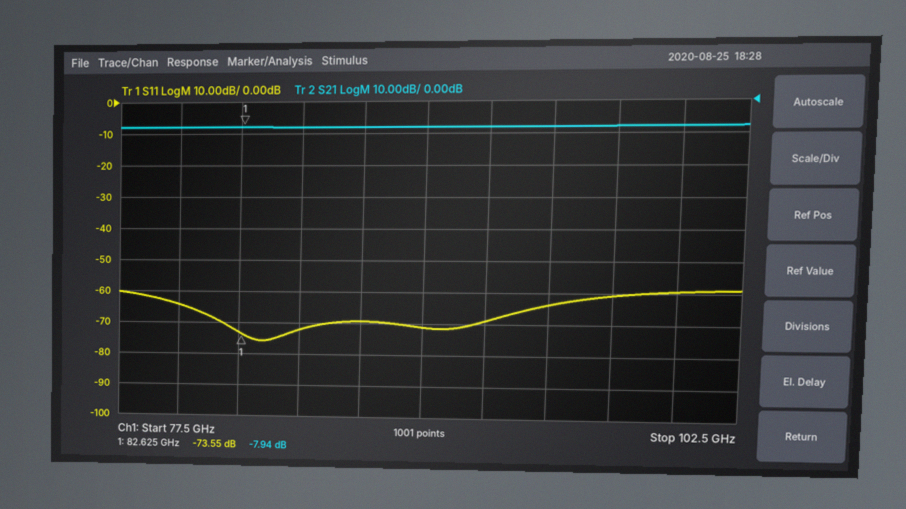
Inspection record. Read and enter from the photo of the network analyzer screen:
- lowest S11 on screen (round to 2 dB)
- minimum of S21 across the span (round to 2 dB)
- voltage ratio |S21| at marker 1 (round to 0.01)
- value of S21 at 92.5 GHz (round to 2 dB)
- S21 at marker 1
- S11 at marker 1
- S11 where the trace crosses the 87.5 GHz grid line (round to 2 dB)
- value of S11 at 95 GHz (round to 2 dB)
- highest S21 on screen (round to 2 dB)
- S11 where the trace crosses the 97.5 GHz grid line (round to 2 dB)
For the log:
-76 dB
-8 dB
0.40
-8 dB
-7.94 dB
-73.55 dB
-70 dB
-64 dB
-8 dB
-60 dB
